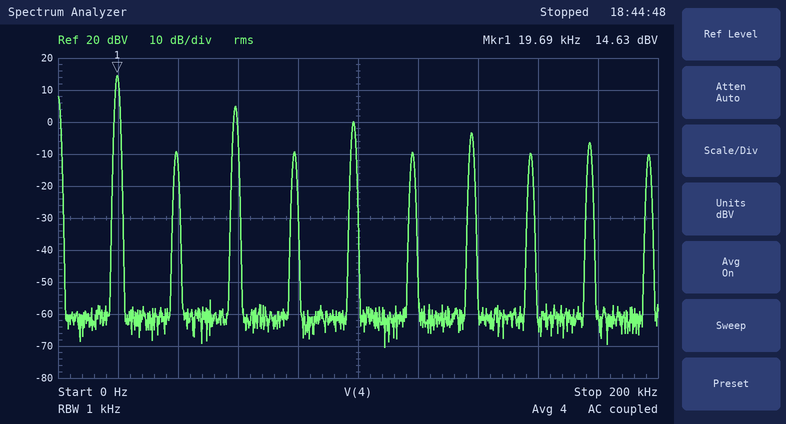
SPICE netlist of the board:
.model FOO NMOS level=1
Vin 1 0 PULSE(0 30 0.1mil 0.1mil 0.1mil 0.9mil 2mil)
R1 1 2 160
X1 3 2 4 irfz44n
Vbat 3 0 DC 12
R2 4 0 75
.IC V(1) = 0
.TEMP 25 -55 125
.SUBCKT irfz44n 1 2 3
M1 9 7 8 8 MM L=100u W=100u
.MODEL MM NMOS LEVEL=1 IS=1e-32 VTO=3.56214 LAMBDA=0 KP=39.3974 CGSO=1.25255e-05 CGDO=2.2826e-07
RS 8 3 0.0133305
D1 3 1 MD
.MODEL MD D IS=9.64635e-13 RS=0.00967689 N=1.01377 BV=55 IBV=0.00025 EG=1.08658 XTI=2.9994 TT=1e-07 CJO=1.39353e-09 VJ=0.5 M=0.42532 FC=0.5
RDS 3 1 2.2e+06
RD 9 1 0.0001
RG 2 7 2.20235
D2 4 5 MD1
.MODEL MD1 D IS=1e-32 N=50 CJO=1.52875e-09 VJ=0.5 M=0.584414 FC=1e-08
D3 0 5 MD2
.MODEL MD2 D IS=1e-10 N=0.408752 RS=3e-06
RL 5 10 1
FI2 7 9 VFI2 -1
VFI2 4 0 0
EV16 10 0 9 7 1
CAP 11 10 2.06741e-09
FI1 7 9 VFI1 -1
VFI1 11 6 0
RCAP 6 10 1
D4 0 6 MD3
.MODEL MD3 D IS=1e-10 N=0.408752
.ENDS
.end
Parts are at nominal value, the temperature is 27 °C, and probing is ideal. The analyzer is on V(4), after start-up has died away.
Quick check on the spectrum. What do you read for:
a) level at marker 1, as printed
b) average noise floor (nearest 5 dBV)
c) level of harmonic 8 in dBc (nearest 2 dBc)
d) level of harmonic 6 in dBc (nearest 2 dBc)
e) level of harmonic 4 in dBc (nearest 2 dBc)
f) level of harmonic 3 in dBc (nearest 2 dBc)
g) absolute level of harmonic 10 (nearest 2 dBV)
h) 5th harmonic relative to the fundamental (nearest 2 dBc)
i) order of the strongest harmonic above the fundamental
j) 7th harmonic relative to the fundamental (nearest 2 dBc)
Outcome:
14.63 dBV
-60 dBV
-24 dBc
-24 dBc
-24 dBc
-10 dBc
-10 dBV
-14 dBc
3
-18 dBc
